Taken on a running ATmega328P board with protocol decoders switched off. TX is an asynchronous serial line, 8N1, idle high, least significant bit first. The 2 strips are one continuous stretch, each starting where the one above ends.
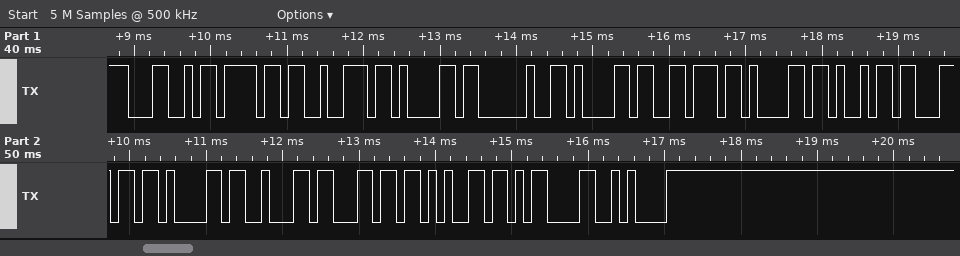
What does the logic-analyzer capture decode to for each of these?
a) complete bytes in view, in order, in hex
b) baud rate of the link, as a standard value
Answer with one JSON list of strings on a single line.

["4C 6F 72 61 20 61 76 61 69 6C 61 62 6C 65 0D 0A", "9600 baud"]
